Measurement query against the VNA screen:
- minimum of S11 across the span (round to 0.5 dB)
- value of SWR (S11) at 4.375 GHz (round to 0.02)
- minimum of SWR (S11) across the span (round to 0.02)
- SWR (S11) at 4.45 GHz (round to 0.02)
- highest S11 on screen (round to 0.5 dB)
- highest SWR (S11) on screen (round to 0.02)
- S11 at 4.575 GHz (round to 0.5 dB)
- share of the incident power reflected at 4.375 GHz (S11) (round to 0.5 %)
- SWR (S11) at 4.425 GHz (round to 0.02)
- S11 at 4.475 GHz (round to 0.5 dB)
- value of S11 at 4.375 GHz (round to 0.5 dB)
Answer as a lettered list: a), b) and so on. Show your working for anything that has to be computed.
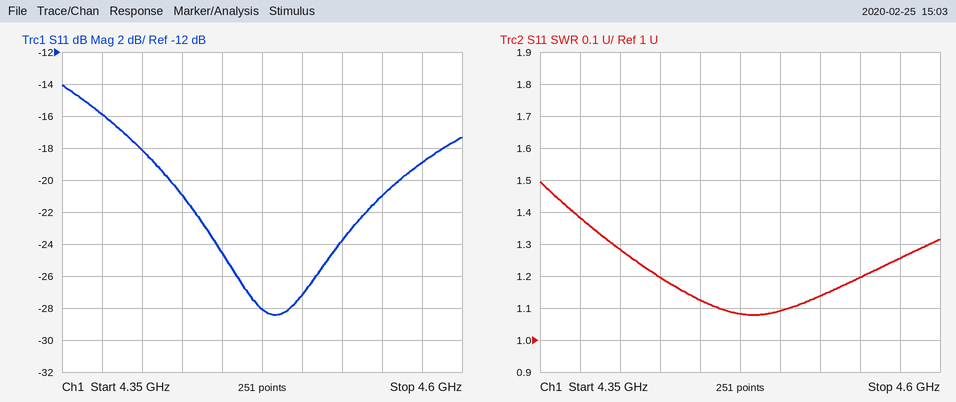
a) -28.5 dB
b) 1.38
c) 1.08
d) 1.12
e) -14.0 dB
f) 1.50
g) -19.0 dB
h) 10^(-16/10) ≈ 2.5 %
i) 1.20
j) -28.0 dB
k) -16.0 dB
